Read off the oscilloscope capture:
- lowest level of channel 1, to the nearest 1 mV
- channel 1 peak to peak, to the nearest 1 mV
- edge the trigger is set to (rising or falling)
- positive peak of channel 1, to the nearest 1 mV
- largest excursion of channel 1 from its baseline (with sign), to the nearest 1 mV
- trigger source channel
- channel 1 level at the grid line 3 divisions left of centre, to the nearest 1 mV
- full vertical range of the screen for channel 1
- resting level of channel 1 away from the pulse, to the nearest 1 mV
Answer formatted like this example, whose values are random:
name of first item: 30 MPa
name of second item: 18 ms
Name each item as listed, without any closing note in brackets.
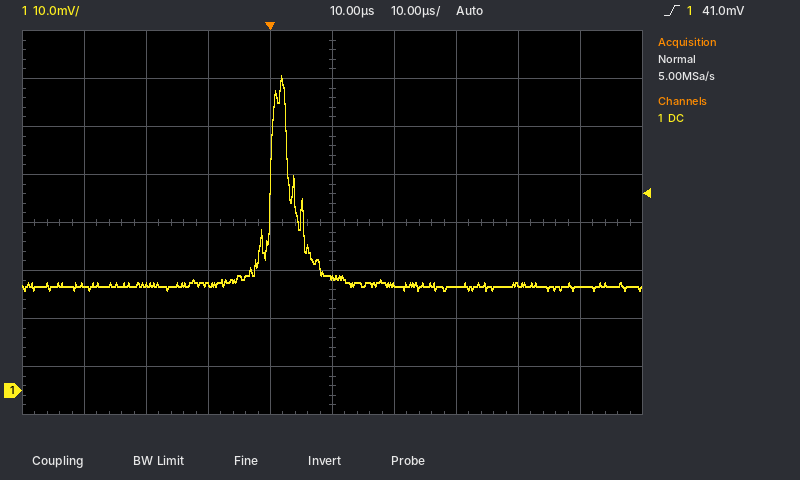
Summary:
lowest level of channel 1, to the nearest 1 mV: 21 mV
channel 1 peak to peak, to the nearest 1 mV: 45 mV
edge the trigger is set to: rising
positive peak of channel 1, to the nearest 1 mV: 66 mV
largest excursion of channel 1 from its baseline (with sign), to the nearest 1 mV: +44 mV
trigger source channel: channel 1
channel 1 level at the grid line 3 divisions left of centre, to the nearest 1 mV: 22 mV
full vertical range of the screen for channel 1: 80 mV
resting level of channel 1 away from the pulse, to the nearest 1 mV: 22 mV
